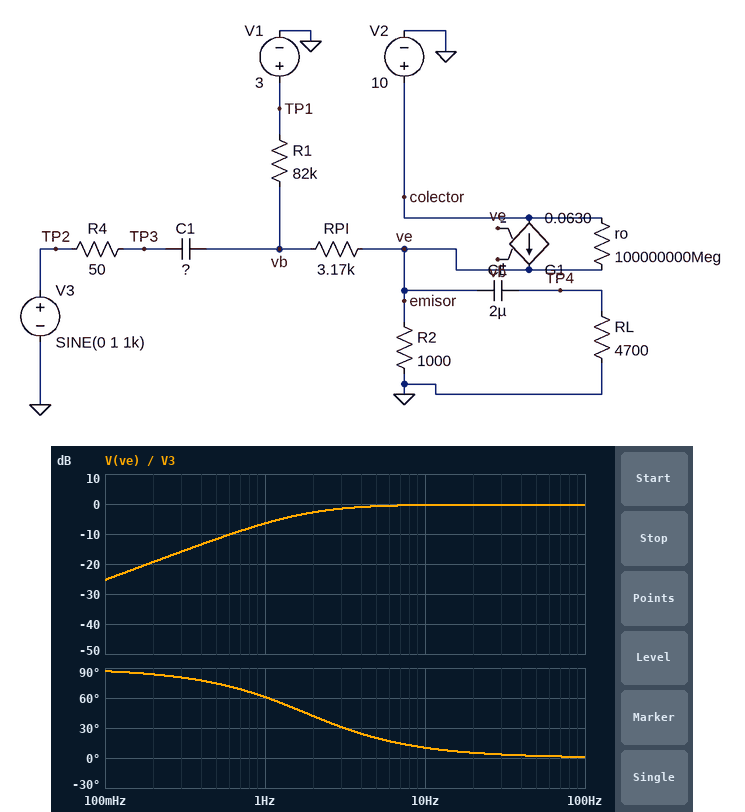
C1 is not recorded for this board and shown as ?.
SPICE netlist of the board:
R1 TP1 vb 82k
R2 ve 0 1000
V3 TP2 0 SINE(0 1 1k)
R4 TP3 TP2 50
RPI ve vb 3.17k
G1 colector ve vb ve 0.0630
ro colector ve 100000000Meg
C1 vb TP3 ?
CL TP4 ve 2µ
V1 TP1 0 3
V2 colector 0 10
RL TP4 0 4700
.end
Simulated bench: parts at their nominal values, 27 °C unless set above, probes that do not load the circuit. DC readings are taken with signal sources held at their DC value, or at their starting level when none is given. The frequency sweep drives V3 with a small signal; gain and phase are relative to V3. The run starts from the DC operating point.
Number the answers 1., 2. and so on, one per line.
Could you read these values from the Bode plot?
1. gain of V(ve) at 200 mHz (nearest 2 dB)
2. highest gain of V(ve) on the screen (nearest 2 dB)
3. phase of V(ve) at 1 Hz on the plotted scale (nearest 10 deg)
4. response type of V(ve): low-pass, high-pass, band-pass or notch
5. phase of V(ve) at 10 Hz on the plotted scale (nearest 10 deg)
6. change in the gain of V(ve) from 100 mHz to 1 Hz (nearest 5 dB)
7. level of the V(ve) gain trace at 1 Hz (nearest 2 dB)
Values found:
1. -20 dB
2. 0 dB
3. 60 deg
4. high-pass
5. 10 deg
6. 20 dB
7. -6 dB
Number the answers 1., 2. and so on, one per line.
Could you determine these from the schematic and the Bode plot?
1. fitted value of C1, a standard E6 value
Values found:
1. 1.5 µF
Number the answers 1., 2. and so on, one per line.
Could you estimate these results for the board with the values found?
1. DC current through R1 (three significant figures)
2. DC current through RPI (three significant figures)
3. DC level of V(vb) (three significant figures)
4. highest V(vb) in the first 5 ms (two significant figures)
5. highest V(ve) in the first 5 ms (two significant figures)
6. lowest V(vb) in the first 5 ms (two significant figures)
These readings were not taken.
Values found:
1. 10.5 µA
2. 10.5 µA
3. 2.14 V
4. 3.1 V
5. 3.1 V
6. 1.1 V
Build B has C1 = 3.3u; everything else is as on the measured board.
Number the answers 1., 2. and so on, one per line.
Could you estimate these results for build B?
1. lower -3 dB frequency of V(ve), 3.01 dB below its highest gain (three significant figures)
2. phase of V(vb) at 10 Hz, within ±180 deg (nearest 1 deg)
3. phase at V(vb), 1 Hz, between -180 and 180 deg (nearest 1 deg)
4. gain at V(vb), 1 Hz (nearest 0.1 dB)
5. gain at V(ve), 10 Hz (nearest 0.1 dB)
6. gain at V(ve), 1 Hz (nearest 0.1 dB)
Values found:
1. 821 mHz
2. 5 deg
3. 39 deg
4. -2.3 dB
5. -0.2 dB
6. -2.4 dB
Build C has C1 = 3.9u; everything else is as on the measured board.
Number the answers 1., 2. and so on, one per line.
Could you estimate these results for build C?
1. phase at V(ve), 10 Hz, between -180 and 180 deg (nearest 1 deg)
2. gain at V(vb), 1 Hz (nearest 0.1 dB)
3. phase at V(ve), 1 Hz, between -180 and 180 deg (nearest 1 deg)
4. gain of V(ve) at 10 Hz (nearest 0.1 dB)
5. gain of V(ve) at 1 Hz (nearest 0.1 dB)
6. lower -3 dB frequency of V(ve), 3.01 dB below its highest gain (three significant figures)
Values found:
1. 4 deg
2. -1.7 dB
3. 35 deg
4. -0.2 dB
5. -1.9 dB
6. 694 mHz
